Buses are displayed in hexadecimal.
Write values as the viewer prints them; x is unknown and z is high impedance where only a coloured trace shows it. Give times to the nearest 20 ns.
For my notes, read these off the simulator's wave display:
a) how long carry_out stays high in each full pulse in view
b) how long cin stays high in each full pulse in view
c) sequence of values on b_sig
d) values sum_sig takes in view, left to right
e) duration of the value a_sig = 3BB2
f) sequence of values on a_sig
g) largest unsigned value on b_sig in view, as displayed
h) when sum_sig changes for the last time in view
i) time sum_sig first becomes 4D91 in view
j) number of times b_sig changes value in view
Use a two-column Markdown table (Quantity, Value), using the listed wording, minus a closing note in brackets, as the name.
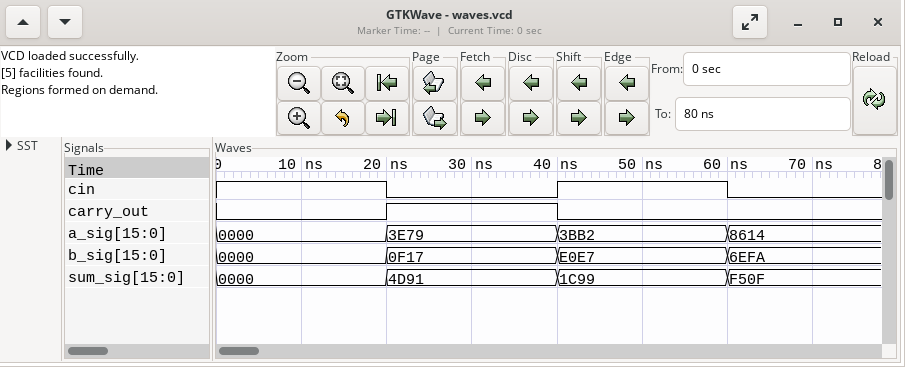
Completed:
| Quantity | Value |
|---|---|
| how long carry_out stays high in each full pulse in view | 20 ns |
| how long cin stays high in each full pulse in view | 20 ns |
| sequence of values on b_sig | 0000, 0F17, E0E7, 6EFA |
| values sum_sig takes in view, left to right | 0000, 4D91, 1C99, F50F |
| duration of the value a_sig = 3BB2 | 20 ns |
| sequence of values on a_sig | 0000, 3E79, 3BB2, 8614 |
| largest unsigned value on b_sig in view, as displayed | E0E7 |
| when sum_sig changes for the last time in view | 60 ns |
| time sum_sig first becomes 4D91 in view | 20 ns |
| number of times b_sig changes value in view | 3 |
